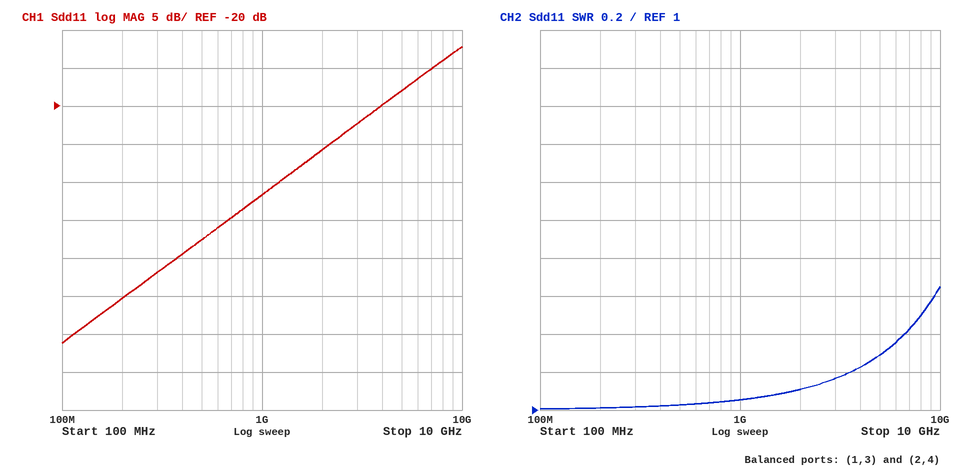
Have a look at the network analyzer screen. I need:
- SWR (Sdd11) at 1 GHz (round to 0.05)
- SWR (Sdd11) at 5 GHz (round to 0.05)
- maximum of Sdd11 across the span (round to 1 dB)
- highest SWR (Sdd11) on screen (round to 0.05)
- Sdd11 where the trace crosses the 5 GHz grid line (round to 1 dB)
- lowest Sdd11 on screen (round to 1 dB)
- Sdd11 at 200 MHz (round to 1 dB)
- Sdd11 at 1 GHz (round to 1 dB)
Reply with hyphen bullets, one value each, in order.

- 1.05
- 1.30
- -12 dB
- 1.65
- -18 dB
- -51 dB
- -45 dB
- -32 dB
